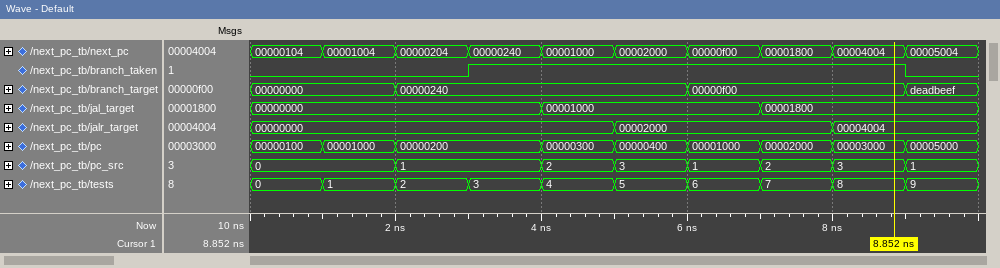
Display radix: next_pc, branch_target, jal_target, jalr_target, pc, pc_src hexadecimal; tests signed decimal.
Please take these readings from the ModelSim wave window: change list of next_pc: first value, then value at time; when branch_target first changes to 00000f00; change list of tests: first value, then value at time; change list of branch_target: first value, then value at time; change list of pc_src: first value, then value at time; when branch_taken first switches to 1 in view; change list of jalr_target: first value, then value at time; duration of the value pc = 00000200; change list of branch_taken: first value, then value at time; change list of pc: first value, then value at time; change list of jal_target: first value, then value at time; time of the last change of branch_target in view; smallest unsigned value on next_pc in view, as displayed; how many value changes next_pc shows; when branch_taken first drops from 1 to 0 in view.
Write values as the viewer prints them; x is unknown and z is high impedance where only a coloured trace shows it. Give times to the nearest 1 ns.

00000104, 00001004 at 1 ns, 00000204 at 2 ns, 00000240 at 3 ns, 00001000 at 4 ns, 00002000 at 5 ns, 00000f00 at 6 ns, 00001800 at 7 ns, 00004004 at 8 ns, 00005004 at 9 ns
6 ns
0, 1 at 1 ns, 2 at 2 ns, 3 at 3 ns, 4 at 4 ns, 5 at 5 ns, 6 at 6 ns, 7 at 7 ns, 8 at 8 ns, 9 at 9 ns
00000000, 00000240 at 2 ns, 00000f00 at 6 ns, deadbeef at 9 ns
0, 1 at 2 ns, 2 at 4 ns, 3 at 5 ns, 1 at 6 ns, 2 at 7 ns, 3 at 8 ns, 1 at 9 ns
3 ns
00000000, 00002000 at 5 ns, 00004004 at 8 ns
2 ns
0, 1 at 3 ns, 0 at 9 ns
00000100, 00001000 at 1 ns, 00000200 at 2 ns, 00000300 at 4 ns, 00000400 at 5 ns, 00001000 at 6 ns, 00002000 at 7 ns, 00003000 at 8 ns, 00005000 at 9 ns
00000000, 00001000 at 4 ns, 00001800 at 7 ns
9 ns
00000104
9
9 ns
